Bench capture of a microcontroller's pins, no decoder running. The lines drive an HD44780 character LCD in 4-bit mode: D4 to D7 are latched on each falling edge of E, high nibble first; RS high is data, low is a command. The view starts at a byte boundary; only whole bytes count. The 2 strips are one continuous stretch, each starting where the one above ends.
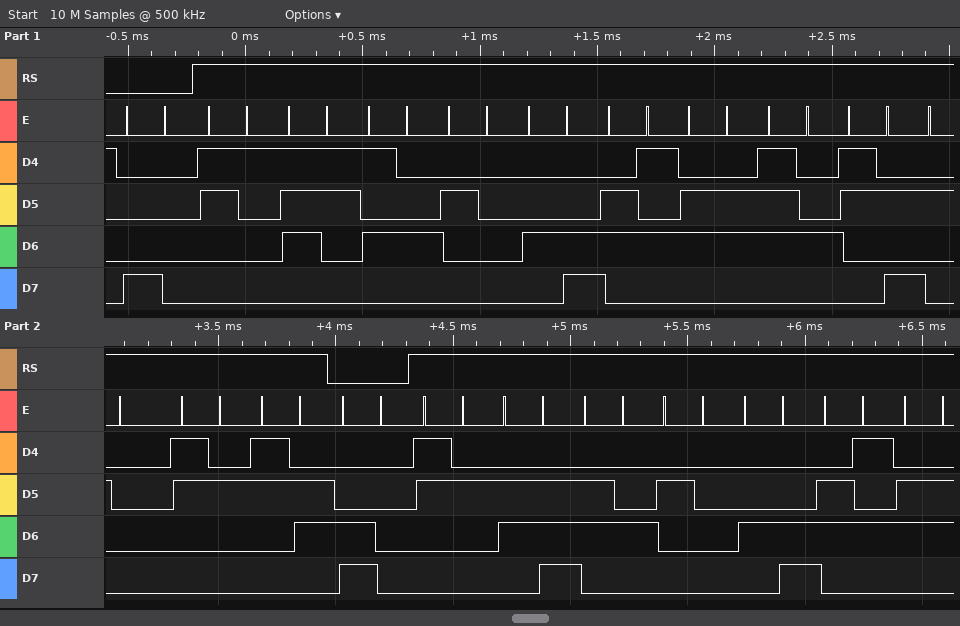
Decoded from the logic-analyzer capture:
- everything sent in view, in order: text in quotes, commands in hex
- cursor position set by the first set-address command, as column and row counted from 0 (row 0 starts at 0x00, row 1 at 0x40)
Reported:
0x80 "1sT Left: 26" 0xC0 "2nd Lef"
column 0, row 0
